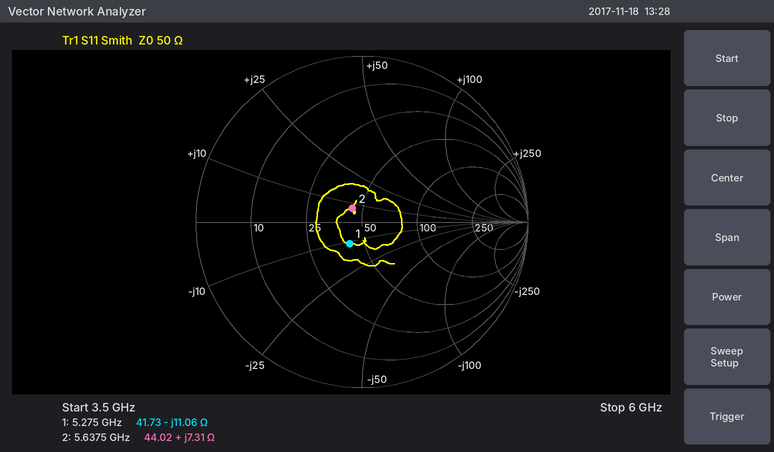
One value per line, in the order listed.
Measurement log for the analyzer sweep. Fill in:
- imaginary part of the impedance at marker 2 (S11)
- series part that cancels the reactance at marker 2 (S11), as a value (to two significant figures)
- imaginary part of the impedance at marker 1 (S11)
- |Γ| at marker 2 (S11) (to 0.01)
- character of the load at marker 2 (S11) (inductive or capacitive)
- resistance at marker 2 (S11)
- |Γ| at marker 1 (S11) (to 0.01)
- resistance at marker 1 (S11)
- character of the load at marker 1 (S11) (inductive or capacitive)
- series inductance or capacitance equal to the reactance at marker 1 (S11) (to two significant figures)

+7.31 Ω
3.9 pF
-11.06 Ω
0.10
inductive
44.02 Ω
0.15
41.73 Ω
capacitive
2.7 pF
